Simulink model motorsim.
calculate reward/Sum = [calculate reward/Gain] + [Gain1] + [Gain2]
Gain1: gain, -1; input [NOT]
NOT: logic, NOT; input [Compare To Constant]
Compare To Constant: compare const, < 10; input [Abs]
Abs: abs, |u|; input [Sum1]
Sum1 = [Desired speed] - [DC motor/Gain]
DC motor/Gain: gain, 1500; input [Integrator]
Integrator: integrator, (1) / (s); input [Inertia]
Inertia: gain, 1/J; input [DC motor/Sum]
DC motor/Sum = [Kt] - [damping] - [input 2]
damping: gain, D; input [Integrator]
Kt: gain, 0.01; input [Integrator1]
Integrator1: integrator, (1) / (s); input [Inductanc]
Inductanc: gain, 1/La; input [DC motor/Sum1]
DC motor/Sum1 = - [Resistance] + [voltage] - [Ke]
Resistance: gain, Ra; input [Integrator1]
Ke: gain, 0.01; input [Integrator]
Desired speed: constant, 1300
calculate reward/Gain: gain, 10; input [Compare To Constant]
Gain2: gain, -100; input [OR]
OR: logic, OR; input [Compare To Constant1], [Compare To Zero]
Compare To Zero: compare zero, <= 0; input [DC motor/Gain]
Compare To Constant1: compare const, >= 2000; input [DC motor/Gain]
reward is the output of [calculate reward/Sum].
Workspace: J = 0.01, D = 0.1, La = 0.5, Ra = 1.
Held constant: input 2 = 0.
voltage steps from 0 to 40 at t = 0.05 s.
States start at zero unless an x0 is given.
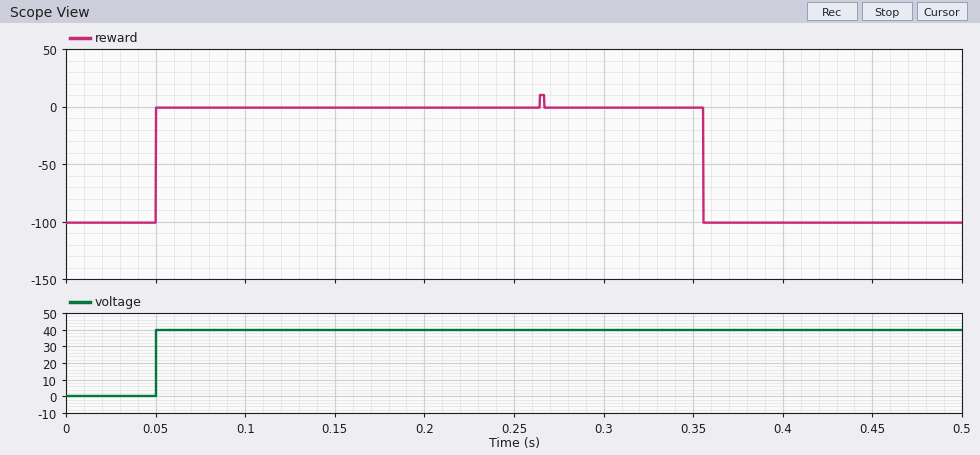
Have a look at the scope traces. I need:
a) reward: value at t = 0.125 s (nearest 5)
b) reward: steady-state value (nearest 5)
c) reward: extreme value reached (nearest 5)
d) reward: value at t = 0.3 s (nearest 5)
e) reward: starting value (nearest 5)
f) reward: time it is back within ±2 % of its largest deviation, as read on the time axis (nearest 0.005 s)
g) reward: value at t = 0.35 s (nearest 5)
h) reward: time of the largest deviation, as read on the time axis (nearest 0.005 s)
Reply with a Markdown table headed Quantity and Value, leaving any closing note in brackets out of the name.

| Quantity | Value |
|---|---|
| reward: value at t = 0.125 s | 0 |
| reward: steady-state value | -100 |
| reward: extreme value reached | 10 |
| reward: value at t = 0.3 s | 0 |
| reward: starting value | -100 |
| reward: time it is back within ±2 % of its largest deviation, as read on the time axis | 0.355 s |
| reward: value at t = 0.35 s | 0 |
| reward: time of the largest deviation, as read on the time axis | 0.265 s |
